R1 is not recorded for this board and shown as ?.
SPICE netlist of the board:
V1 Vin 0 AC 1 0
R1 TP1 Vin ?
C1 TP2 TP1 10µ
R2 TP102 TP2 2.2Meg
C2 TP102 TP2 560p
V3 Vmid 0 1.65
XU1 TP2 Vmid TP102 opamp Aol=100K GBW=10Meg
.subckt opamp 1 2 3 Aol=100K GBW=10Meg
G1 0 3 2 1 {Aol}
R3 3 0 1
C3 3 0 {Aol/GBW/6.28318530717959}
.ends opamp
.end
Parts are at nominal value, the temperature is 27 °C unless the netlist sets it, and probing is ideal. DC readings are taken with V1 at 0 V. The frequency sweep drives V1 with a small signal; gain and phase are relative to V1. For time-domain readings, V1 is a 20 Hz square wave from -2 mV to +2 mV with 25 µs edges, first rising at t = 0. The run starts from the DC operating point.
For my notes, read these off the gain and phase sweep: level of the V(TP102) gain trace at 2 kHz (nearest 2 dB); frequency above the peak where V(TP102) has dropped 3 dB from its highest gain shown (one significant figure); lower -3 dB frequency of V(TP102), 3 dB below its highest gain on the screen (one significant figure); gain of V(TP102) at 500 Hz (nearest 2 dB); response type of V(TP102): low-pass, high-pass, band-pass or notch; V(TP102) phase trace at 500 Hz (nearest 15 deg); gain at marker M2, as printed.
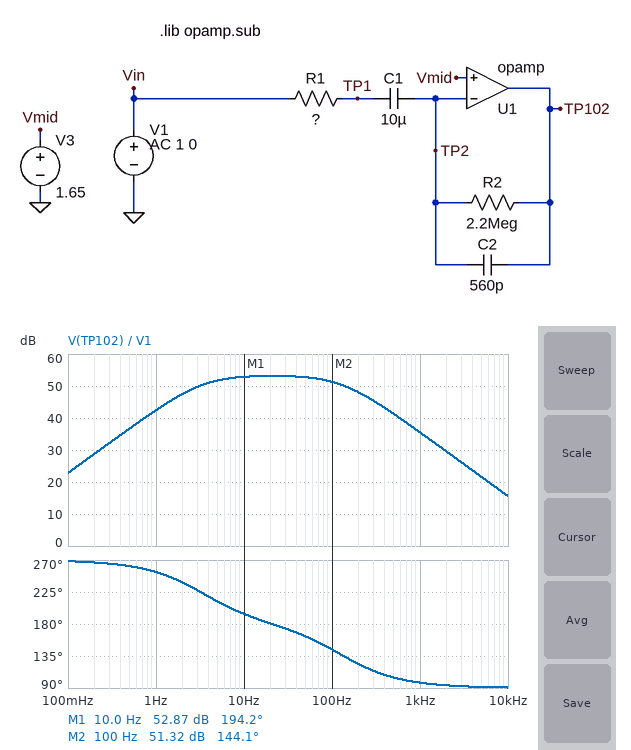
30 dB
100 Hz
3 Hz
42 dB
band-pass
105 deg
51.32 dB
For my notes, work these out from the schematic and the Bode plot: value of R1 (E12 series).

4.7 kΩ
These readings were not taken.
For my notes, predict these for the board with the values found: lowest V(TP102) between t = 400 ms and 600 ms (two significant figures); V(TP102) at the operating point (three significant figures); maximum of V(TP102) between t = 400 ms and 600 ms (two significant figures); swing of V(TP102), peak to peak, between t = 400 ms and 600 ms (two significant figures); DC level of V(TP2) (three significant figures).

600 mV
1.65 V
2.7 V
2.1 V
1.65 V
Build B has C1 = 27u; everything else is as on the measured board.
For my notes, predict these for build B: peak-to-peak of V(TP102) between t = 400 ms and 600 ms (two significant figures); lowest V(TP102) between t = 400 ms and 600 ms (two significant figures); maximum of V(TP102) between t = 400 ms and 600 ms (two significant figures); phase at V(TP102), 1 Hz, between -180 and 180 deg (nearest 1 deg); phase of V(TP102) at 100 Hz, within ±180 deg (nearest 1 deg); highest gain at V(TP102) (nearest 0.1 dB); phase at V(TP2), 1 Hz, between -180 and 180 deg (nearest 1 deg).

2.0 V
640 mV
2.6 V
-129 deg
143 deg
53.3 dB
51 deg
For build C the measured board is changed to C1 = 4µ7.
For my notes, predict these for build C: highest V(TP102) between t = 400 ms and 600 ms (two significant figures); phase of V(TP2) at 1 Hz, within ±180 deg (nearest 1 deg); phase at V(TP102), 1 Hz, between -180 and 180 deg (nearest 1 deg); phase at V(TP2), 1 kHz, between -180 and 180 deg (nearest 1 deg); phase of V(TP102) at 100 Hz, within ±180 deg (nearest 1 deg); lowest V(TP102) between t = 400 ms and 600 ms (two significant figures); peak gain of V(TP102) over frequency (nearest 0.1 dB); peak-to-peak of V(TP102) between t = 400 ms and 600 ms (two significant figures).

2.8 V
82 deg
-98 deg
2 deg
146 deg
480 mV
52.9 dB
2.3 V
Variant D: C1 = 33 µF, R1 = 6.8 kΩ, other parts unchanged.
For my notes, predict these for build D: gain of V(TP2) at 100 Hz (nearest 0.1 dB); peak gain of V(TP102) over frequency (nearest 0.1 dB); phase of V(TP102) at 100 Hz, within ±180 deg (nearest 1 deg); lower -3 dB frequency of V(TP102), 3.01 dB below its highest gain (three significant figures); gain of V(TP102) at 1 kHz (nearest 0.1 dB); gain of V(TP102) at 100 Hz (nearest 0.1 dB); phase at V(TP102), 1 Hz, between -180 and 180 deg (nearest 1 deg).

-48.9 dB
50.1 dB
143 deg
699 mHz
32.3 dB
48.1 dB
-145 deg
